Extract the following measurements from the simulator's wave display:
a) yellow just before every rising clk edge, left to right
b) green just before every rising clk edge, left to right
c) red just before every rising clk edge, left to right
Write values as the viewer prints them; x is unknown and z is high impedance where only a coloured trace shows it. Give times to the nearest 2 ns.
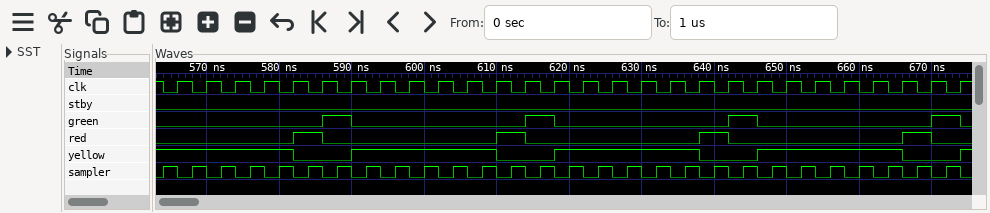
1 1 1 1 1 0 0 1 1 1 1 1 0 0 1 1 1 1 1 0 0 1 1 1 1 1 0 0
0 0 0 0 0 0 1 0 0 0 0 0 0 1 0 0 0 0 0 0 1 0 0 0 0 0 0 1
0 0 0 0 0 1 0 0 0 0 0 0 1 0 0 0 0 0 0 1 0 0 0 0 0 0 1 0
